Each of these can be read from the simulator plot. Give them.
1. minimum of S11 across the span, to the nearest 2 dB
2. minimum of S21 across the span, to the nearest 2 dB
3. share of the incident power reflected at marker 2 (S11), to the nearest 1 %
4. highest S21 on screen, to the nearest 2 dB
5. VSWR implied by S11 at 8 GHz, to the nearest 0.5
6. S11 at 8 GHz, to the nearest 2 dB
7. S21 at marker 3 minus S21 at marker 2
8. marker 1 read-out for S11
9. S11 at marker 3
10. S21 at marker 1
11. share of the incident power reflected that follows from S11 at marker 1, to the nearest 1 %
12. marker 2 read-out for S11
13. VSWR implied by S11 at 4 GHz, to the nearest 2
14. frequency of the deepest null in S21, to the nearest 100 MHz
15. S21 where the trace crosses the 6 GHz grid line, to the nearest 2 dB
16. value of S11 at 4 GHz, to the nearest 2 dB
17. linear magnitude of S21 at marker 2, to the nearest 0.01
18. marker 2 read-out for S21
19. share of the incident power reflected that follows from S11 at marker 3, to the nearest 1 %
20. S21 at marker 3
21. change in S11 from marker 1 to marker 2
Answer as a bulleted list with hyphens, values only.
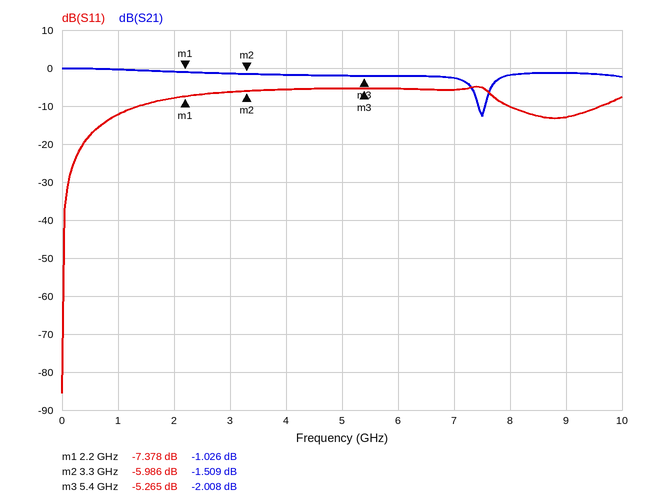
- -86 dB
- -12 dB
- 25 %
- 0 dB
- 2.0
- -10 dB
- -0.499 dB
- -7.378 dB
- -5.265 dB
- -1.026 dB
- 18 %
- -5.986 dB
- 4
- 7.5 GHz
- -2 dB
- -6 dB
- 0.84
- -1.509 dB
- 30 %
- -2.008 dB
- 1.392 dB
